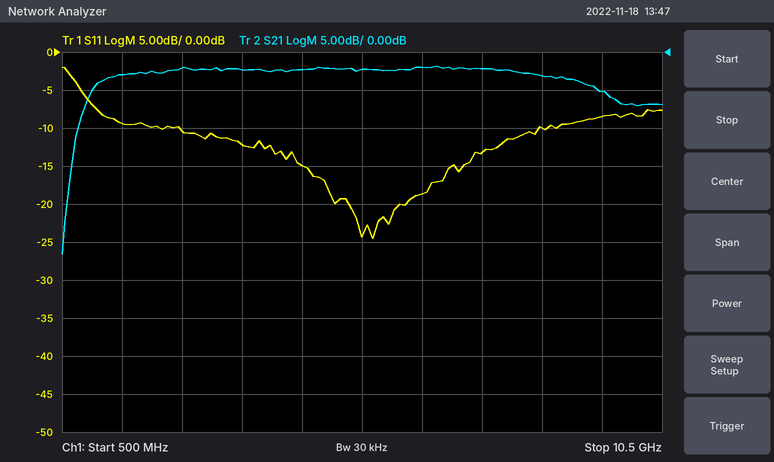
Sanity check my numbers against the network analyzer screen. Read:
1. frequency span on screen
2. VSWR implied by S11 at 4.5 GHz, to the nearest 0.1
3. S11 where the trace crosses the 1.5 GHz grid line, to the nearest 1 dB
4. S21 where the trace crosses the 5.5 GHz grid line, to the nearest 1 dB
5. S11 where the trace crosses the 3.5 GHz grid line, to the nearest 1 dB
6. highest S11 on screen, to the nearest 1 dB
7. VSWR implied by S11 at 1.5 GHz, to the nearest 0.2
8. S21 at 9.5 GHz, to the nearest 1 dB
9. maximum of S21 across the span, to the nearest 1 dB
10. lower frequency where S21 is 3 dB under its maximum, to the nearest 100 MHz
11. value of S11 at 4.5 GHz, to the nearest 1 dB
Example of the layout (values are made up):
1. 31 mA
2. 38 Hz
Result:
1. 10 GHz
2. 1.4
3. -9 dB
4. -2 dB
5. -12 dB
6. -2 dB
7. 2.0
8. -5 dB
9. -2 dB
10. 1.0 GHz
11. -15 dB
